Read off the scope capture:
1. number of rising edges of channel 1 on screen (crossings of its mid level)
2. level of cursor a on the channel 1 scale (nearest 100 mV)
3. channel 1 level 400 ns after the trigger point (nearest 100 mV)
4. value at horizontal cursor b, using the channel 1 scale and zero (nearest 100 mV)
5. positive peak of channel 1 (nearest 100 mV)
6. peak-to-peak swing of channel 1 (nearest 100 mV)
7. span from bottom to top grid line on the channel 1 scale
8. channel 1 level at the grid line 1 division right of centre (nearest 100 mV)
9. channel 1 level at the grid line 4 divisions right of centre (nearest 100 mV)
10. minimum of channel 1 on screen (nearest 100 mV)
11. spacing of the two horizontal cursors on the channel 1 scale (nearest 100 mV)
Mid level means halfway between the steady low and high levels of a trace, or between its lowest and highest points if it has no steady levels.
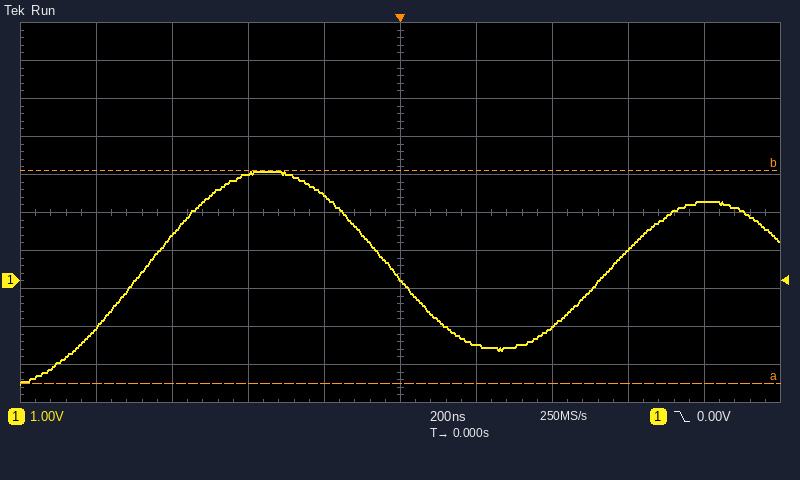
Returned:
2
-2.7 V
-1.2 V
2.9 V
2.9 V
5.6 V
10 V
-1.7 V
2.1 V
-2.7 V
5.6 V
